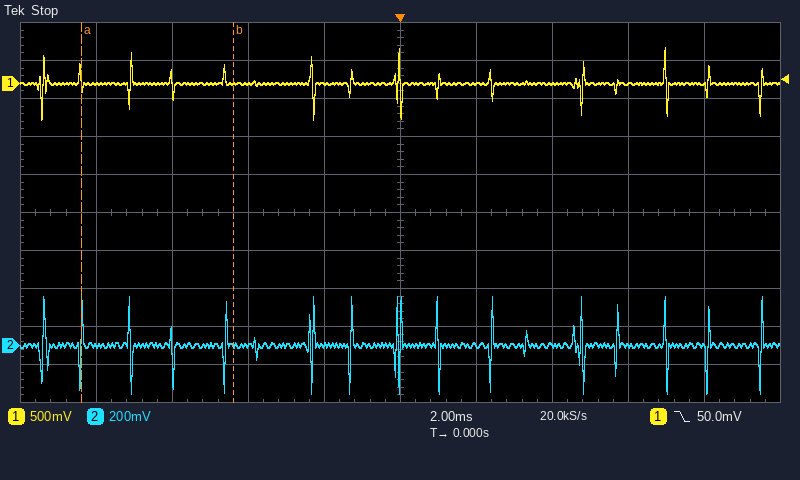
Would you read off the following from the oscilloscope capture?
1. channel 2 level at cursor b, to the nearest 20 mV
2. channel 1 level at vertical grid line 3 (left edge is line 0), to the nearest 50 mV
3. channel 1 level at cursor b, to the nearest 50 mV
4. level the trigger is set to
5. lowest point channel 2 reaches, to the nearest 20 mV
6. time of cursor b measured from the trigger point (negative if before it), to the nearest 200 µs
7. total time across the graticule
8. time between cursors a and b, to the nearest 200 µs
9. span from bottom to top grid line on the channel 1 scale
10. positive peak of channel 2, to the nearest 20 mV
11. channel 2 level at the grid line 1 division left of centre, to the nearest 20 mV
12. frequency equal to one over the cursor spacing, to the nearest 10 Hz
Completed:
0 mV
0 mV
0 mV
50.0 mV
-260 mV
-4.4 ms
20 ms
4.0 ms
5 V
260 mV
0 mV
250 Hz
